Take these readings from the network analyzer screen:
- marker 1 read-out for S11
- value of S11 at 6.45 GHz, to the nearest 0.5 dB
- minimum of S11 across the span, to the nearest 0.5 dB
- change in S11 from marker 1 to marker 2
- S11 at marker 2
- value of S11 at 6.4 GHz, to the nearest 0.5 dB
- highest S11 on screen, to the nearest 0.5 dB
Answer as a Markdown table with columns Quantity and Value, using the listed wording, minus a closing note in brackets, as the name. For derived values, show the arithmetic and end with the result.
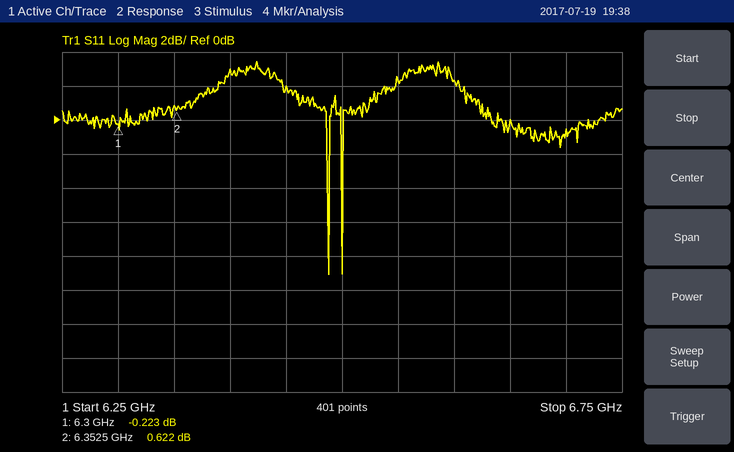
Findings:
| Quantity | Value |
|---|---|
| marker 1 read-out for S11 | -0.223 dB |
| value of S11 at 6.45 GHz, to the nearest 0.5 dB | 2.0 dB |
| minimum of S11 across the span, to the nearest 0.5 dB | -9.0 dB |
| change in S11 from marker 1 to marker 2 | 0.622 − (-0.223) = 0.845 dB |
| S11 at marker 2 | 0.622 dB |
| value of S11 at 6.4 GHz, to the nearest 0.5 dB | 3.0 dB |
| highest S11 on screen, to the nearest 0.5 dB | 3.5 dB |
